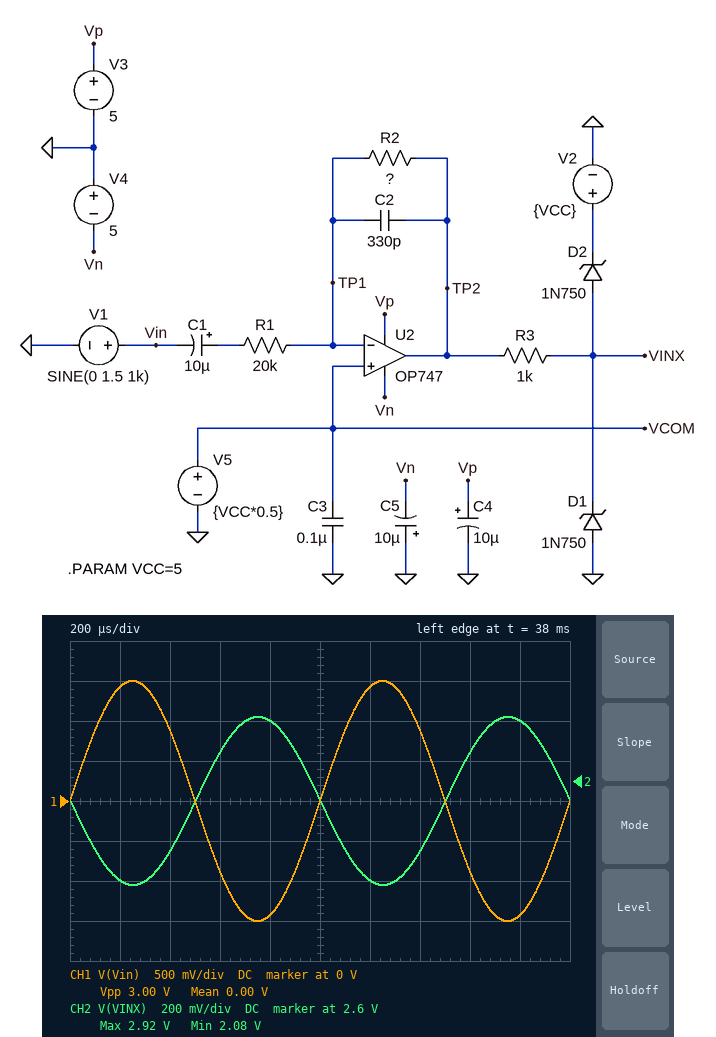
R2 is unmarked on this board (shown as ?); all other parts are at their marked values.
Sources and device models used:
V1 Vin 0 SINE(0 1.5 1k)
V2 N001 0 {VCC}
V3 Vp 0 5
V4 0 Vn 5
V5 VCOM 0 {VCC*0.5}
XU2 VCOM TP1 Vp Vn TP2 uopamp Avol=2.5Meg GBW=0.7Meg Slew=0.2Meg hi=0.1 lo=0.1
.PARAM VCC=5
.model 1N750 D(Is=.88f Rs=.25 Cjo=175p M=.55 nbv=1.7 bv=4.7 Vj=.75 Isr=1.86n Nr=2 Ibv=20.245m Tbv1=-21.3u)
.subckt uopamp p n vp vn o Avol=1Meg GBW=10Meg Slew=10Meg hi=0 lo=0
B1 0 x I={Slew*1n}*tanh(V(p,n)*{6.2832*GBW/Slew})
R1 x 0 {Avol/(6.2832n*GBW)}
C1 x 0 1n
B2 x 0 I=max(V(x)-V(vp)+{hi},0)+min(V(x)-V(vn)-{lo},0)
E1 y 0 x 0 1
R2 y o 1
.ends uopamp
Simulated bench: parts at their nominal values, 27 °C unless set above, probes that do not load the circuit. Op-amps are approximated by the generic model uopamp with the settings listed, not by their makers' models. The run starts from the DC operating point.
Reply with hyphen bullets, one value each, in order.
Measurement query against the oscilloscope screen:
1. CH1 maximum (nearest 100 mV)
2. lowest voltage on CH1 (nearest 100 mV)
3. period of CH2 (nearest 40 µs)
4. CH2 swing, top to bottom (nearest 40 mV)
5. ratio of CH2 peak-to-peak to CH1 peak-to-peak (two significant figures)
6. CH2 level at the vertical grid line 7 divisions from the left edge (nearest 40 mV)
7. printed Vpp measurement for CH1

- 1.5 V
- -1.5 V
- 1.00 ms
- 840 mV
- 0.28
- 2.24 V
- 3.00 V
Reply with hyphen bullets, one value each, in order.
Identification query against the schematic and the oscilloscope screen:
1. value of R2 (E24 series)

- 5.6 kΩ
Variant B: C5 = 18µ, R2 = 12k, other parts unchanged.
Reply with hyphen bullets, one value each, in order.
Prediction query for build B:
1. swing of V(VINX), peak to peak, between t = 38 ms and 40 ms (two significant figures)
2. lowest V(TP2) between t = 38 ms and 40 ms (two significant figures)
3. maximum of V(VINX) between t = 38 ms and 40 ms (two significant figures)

- 1.8 V
- 1.6 V
- 3.4 V
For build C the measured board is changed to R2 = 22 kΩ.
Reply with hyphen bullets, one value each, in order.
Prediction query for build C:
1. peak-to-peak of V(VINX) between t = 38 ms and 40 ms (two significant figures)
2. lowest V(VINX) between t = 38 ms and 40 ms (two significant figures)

- 3.3 V
- 850 mV
